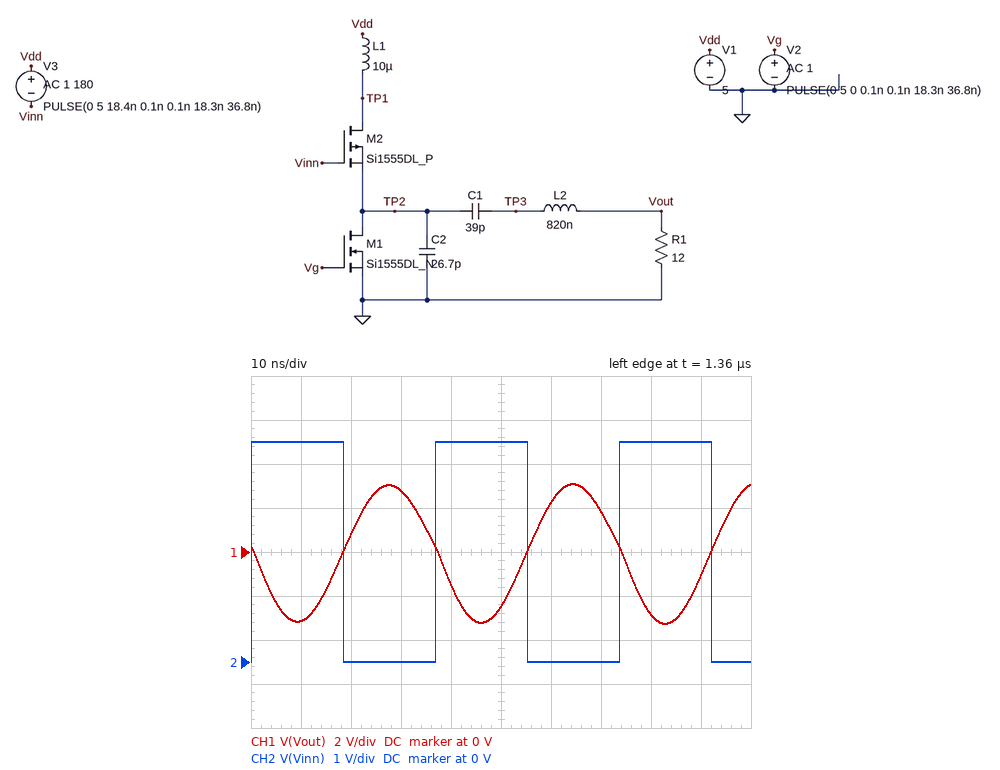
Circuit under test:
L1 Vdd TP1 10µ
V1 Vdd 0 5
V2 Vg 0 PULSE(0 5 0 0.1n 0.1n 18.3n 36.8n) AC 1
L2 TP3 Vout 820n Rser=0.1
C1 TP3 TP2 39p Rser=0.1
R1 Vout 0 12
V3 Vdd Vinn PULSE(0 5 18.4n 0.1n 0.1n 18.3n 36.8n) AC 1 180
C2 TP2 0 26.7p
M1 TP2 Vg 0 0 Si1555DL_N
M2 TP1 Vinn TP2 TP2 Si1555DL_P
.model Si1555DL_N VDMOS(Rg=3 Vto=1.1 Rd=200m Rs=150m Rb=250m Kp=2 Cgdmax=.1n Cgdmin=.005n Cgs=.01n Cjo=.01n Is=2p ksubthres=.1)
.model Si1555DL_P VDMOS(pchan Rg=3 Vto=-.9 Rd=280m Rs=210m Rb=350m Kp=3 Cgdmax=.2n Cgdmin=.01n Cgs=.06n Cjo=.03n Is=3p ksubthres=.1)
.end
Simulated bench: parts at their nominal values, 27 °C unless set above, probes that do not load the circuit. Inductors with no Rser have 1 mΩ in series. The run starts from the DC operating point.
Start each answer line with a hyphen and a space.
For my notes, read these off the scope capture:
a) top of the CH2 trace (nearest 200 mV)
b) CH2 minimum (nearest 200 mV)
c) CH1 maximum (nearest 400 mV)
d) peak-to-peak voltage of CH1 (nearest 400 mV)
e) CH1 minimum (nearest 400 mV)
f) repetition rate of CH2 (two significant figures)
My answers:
- 5.0 V
- 0 V
- 3.2 V
- 6.4 V
- -3.2 V
- 27 MHz
